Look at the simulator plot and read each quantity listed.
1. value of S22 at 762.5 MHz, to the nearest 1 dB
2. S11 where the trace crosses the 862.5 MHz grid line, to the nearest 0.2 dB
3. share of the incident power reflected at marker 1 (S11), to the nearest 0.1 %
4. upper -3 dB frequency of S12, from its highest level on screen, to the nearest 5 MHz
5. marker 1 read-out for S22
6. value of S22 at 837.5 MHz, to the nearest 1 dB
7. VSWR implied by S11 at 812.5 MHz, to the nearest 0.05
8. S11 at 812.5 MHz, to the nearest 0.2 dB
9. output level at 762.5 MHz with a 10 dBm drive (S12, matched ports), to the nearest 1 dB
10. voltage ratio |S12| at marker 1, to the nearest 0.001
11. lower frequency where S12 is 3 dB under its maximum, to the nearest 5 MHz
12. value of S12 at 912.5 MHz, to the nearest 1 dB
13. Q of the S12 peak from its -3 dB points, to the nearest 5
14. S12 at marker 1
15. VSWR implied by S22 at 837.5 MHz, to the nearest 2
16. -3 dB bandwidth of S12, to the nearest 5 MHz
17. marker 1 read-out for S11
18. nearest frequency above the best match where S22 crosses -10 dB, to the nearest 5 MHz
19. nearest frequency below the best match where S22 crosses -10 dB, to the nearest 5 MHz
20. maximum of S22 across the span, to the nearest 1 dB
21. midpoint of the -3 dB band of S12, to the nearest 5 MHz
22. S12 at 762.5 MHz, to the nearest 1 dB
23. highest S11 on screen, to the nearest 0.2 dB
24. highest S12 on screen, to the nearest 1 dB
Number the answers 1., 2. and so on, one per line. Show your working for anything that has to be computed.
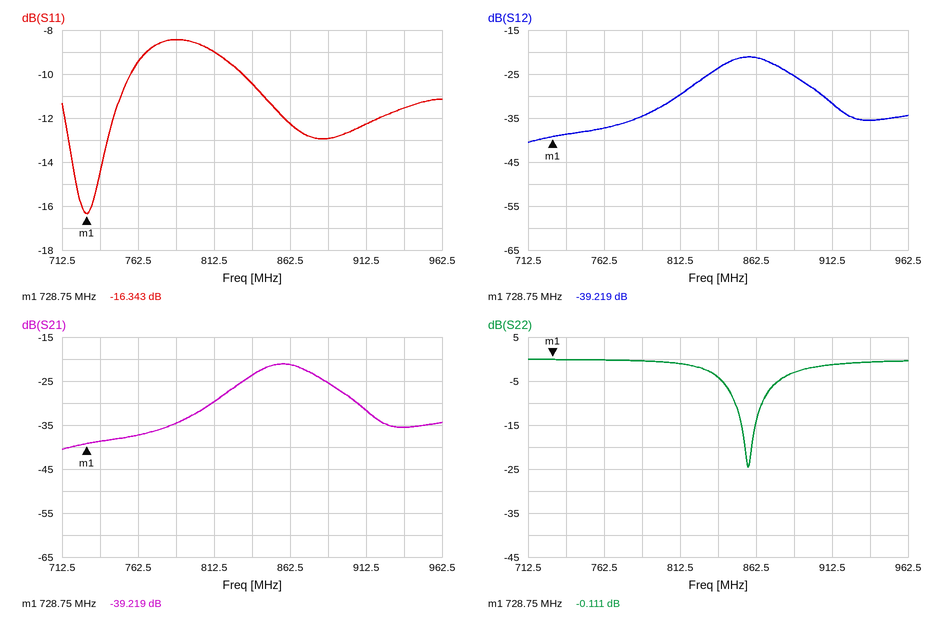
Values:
1. 0 dB
2. -12.2 dB
3. 10^(-16.343/10) ≈ 2.3 %
4. 880 MHz
5. -0.111 dB
6. -4 dB
7. |Γ| = 10^(-9/20) = 0.3548; VSWR = (1 + 0.3548)/(1 − 0.3548) ≈ 2.10
8. -9.0 dB
9. 10 dBm + (-37 dB) = -27 dBm
10. 10^(-39.219/20) ≈ 0.011
11. 835 MHz
12. -32 dB
13. 857.5 MHz / 45 MHz ≈ 19.1, so 20 to the nearest 5
14. -39.219 dB
15. |Γ| = 10^(-4/20) = 0.6310; VSWR = (1 + 0.6310)/(1 − 0.6310) ≈ 4
16. 880 MHz − 835 MHz = 45 MHz
17. -16.343 dB
18. 865 MHz
19. 850 MHz
20. 0 dB
21. 860 MHz
22. -37 dB
23. -8.4 dB
24. -21 dB
